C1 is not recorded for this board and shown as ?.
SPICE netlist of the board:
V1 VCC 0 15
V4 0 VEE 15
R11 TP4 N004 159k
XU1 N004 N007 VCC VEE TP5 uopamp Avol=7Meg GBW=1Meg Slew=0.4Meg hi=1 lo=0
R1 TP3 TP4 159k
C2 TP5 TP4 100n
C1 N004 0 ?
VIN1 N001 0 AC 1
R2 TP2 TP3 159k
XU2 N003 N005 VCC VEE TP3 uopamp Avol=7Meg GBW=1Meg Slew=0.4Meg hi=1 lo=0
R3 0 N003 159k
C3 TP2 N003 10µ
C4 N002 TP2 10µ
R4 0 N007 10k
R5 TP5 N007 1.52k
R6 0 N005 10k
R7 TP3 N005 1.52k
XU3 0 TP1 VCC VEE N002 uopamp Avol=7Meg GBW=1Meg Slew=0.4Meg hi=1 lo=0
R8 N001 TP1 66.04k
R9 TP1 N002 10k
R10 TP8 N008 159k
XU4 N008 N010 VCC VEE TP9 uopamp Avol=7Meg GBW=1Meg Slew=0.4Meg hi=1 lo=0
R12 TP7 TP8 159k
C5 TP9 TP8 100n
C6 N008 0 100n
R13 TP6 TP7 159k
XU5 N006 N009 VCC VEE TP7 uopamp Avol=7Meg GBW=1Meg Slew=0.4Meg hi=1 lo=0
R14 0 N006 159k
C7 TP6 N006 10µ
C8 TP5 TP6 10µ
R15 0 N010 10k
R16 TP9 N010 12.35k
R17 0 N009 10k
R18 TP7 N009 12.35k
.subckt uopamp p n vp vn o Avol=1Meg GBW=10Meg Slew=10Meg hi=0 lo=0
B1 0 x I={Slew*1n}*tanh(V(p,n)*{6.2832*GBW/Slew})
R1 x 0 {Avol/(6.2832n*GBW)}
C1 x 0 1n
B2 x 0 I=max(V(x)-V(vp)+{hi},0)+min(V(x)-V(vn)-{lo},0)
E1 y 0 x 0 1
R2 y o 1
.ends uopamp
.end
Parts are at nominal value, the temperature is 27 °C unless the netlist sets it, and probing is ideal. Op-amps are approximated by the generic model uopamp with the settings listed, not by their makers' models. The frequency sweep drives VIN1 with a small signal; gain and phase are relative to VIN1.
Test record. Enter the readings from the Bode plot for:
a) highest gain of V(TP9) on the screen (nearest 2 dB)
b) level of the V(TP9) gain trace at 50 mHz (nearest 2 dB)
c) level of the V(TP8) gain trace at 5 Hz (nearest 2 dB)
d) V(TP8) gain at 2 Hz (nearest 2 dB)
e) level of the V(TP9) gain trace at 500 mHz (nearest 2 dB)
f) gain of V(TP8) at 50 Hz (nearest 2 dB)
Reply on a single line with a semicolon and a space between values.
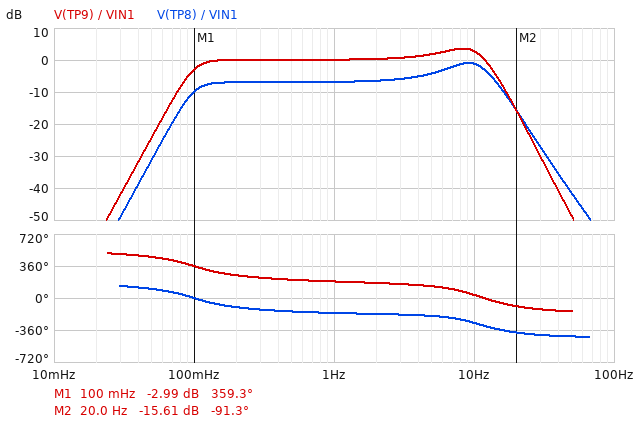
4 dB; -24 dB; -4 dB; -6 dB; 0 dB; -42 dB
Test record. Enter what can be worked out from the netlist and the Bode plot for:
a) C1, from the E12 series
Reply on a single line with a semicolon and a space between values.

47 nF
